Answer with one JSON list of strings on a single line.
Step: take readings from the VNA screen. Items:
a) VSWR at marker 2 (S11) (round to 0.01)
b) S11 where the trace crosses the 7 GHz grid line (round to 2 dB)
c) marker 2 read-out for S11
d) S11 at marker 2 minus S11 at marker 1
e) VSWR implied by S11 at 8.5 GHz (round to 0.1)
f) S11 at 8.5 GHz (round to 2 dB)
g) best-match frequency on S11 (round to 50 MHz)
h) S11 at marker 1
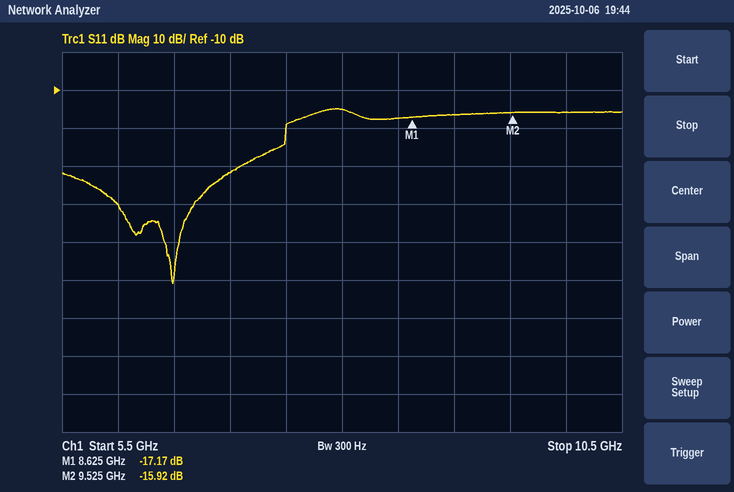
["1.38", "-32 dB", "-15.92 dB", "1.25 dB", "1.3", "-18 dB", "6.50 GHz", "-17.17 dB"]
